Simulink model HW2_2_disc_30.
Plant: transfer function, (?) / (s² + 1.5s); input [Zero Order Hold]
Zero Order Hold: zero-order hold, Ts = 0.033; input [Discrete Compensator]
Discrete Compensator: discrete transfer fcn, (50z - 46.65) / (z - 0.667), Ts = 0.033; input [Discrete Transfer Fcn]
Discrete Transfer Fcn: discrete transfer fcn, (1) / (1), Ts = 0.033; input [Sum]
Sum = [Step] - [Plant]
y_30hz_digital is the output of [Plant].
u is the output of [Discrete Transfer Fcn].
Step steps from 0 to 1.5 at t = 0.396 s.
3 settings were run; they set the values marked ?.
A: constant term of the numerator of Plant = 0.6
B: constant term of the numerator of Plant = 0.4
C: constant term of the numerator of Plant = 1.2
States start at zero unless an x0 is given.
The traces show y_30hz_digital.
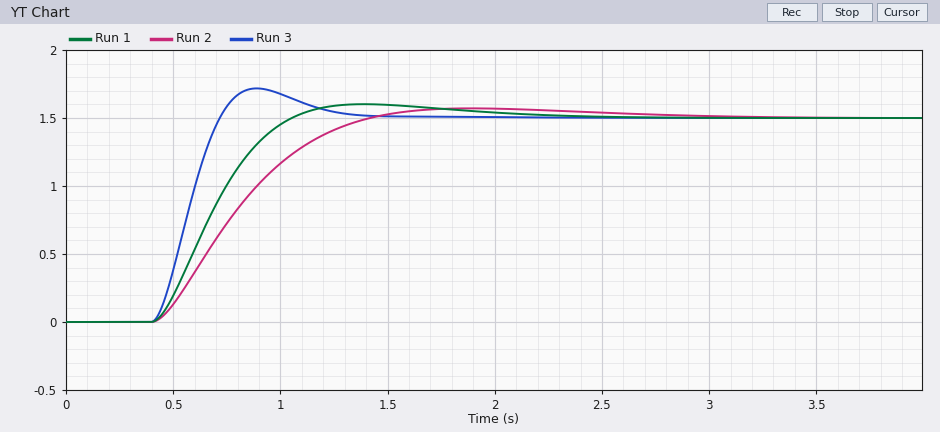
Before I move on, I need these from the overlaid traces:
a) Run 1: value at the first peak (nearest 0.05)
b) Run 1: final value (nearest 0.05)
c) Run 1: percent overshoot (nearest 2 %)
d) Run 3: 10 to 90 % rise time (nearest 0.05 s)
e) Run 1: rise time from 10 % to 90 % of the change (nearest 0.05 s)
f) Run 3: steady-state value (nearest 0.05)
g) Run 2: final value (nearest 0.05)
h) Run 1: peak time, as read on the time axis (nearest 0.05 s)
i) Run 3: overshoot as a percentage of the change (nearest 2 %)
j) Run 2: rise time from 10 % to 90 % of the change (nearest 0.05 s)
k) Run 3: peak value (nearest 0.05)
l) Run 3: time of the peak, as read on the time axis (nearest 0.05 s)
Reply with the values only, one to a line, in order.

1.60
1.50
6 %
0.20 s
0.45 s
1.50
1.50
1.40 s
14 %
0.65 s
1.70
0.90 s
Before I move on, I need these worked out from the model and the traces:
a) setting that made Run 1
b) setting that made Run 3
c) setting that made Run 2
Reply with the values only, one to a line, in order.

A
C
B
